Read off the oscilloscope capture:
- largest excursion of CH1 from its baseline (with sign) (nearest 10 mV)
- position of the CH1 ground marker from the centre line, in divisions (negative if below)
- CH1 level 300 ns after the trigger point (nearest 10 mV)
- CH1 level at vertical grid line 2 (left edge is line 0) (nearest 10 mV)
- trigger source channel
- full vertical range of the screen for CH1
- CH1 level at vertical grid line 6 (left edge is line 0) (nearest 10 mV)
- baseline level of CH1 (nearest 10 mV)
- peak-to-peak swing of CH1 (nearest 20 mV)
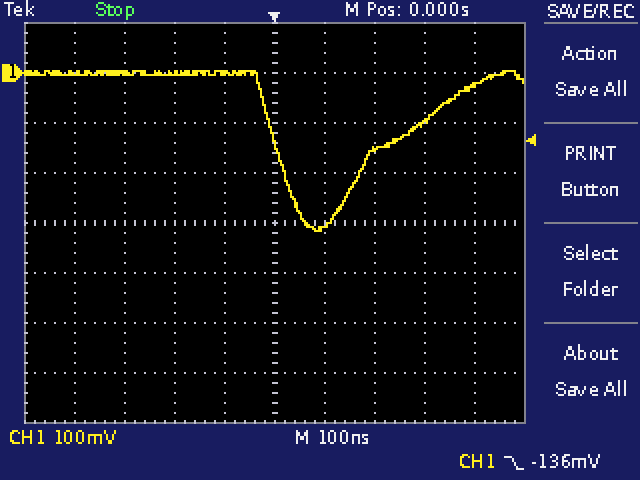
-320 mV
+3.0 div
-100 mV
0 mV
CH1
800 mV
-310 mV
0 mV
320 mV
